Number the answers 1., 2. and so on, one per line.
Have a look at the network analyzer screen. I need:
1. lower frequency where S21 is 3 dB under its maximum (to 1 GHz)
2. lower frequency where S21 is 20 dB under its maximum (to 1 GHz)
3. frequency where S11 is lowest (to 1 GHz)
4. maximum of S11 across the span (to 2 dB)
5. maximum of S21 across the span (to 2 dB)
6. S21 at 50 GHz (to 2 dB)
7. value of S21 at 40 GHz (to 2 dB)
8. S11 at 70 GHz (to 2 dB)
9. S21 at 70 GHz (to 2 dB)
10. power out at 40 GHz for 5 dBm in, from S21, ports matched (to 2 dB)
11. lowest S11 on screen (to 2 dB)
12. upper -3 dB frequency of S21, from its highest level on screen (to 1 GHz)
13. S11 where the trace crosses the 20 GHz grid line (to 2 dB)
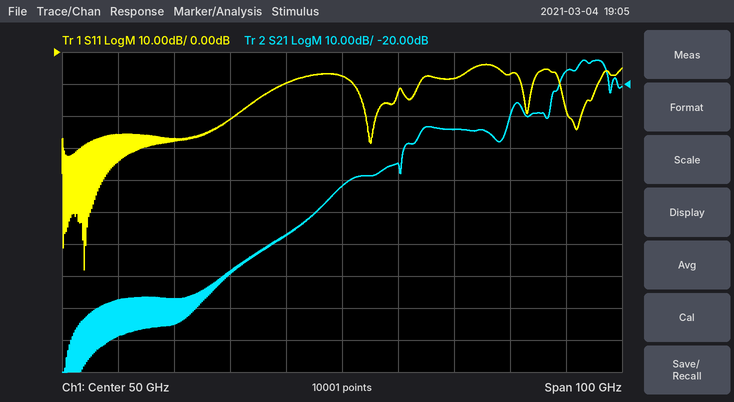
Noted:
1. 92 GHz
2. 80 GHz
3. 4 GHz
4. -4 dB
5. -12 dB
6. -52 dB
7. -68 dB
8. -8 dB
9. -34 dB
10. -62 dBm
11. -68 dB
12. 97 GHz
13. -28 dB
